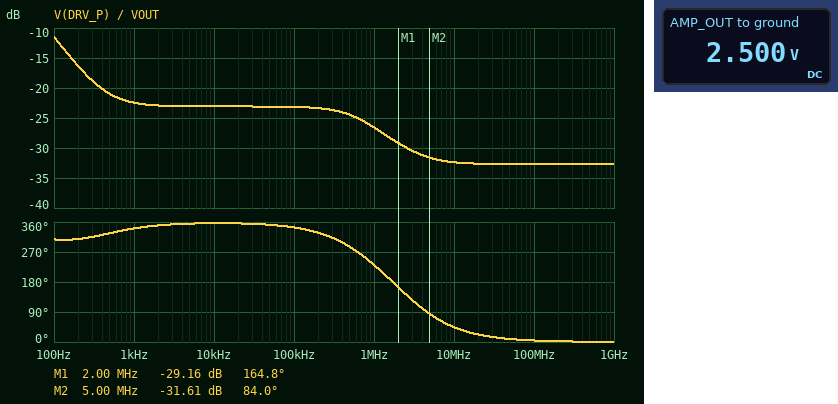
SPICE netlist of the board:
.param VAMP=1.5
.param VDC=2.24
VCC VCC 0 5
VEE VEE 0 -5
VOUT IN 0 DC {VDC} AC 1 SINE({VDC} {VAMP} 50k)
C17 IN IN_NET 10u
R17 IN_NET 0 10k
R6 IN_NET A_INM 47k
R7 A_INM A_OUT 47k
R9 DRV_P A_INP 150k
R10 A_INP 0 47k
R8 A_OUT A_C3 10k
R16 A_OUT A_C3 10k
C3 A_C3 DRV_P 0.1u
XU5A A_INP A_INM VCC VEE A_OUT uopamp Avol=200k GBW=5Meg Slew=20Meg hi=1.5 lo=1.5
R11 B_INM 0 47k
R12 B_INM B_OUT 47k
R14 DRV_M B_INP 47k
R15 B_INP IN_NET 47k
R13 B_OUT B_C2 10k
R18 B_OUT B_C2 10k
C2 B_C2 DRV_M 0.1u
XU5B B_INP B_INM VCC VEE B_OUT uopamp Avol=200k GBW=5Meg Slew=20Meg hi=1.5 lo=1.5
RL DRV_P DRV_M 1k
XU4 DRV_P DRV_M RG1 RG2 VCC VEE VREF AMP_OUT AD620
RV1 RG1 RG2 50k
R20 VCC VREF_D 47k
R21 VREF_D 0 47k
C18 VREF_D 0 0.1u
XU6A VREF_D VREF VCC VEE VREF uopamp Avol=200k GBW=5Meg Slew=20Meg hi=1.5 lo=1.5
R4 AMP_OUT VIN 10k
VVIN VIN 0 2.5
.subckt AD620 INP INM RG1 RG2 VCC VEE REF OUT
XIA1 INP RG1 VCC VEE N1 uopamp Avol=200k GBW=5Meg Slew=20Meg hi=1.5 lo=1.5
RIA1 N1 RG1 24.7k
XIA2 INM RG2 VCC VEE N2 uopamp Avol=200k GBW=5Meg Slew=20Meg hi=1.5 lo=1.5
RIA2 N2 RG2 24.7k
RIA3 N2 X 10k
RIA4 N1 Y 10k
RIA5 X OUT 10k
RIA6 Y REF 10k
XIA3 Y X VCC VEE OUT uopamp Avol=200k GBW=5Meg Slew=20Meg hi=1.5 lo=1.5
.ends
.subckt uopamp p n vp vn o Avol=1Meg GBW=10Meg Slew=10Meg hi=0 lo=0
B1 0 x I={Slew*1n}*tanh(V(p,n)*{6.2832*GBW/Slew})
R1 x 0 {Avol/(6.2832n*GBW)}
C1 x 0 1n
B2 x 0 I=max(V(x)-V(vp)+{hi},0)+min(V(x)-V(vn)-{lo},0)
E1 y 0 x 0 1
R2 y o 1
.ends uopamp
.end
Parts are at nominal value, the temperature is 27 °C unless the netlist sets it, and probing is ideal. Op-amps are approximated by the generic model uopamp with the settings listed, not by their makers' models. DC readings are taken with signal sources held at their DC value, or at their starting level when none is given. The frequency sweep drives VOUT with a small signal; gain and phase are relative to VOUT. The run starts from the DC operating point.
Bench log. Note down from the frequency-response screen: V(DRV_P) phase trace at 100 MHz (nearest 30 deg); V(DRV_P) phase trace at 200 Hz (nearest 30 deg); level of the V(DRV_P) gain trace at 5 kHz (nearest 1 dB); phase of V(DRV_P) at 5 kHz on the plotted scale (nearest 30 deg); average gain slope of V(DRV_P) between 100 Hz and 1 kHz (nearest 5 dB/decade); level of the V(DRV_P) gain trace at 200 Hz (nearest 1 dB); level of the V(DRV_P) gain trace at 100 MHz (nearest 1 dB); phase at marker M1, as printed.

0 deg
300 deg
-23 dB
360 deg
-10 dB/decade
-16 dB
-33 dB
164.8 deg
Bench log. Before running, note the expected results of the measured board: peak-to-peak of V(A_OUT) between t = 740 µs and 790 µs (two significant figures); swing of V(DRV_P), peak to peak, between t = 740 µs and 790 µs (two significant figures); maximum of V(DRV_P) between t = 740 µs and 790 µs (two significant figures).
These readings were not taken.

2.9 V
210 mV
110 mV
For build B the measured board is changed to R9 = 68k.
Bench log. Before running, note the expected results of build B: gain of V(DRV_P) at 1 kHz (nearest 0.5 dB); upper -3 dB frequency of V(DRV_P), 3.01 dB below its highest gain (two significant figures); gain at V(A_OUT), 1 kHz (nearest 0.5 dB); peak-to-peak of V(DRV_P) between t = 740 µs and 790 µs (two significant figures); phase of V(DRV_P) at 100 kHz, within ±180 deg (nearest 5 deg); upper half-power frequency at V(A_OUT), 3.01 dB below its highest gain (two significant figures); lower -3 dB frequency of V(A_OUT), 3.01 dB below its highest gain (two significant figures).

-16.0 dB
120 Hz
-1.0 dB
450 mV
-25 deg
2.6 MHz
91 Hz
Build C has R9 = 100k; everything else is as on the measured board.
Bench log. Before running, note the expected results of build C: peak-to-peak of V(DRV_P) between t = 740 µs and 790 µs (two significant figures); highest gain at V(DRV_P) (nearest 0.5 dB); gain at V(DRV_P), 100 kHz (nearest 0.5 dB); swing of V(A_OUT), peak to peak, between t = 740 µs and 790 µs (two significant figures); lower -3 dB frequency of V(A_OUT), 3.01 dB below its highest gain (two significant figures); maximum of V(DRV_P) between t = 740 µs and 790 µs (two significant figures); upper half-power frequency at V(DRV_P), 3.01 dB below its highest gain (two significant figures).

280 mV
-4.5 dB
-20.5 dB
2.8 V
32 Hz
140 mV
67 Hz
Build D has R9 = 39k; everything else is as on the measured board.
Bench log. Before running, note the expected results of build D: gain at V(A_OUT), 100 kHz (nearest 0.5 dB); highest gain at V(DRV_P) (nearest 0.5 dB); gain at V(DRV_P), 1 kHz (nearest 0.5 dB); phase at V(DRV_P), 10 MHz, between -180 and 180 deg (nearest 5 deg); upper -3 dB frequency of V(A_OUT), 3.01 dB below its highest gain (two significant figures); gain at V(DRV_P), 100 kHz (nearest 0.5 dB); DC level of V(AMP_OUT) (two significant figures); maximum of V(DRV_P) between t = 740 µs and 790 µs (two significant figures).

1.0 dB
7.5 dB
1.5 dB
40 deg
70 kHz
-6.0 dB
2.5 V
1.4 V
